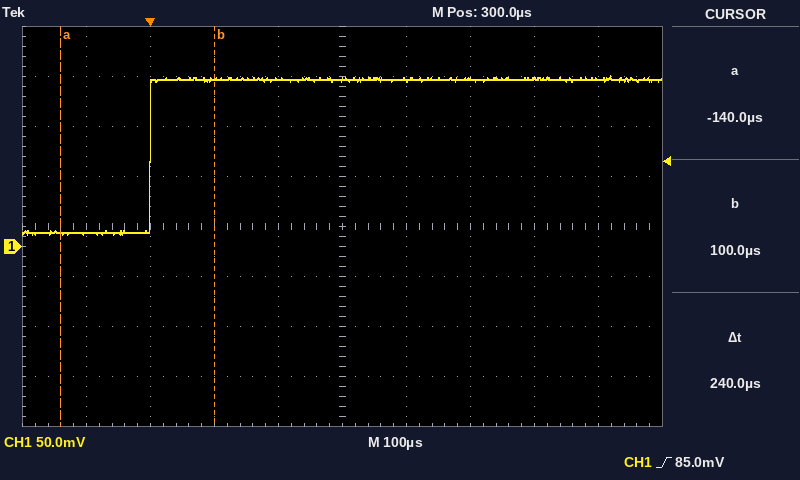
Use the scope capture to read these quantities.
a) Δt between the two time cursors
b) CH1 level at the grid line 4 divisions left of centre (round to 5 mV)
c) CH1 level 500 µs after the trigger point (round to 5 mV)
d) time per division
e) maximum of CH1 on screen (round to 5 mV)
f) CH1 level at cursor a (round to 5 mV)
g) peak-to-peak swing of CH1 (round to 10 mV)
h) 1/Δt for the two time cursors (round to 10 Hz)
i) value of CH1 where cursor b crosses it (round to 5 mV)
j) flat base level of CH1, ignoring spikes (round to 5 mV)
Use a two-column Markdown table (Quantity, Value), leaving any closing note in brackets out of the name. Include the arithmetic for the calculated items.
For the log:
| Quantity | Value |
|---|---|
| Δt between the two time cursors | 240 µs |
| CH1 level at the grid line 4 divisions left of centre | 15 mV |
| CH1 level 500 µs after the trigger point | 170 mV |
| time per division | 100 µs |
| maximum of CH1 on screen | 170 mV |
| CH1 level at cursor a | 15 mV |
| peak-to-peak swing of CH1 | 160 mV |
| 1/Δt for the two time cursors | 1 / 240 µs ≈ 4.17 kHz |
| value of CH1 where cursor b crosses it | 170 mV |
| flat base level of CH1, ignoring spikes | 15 mV |
